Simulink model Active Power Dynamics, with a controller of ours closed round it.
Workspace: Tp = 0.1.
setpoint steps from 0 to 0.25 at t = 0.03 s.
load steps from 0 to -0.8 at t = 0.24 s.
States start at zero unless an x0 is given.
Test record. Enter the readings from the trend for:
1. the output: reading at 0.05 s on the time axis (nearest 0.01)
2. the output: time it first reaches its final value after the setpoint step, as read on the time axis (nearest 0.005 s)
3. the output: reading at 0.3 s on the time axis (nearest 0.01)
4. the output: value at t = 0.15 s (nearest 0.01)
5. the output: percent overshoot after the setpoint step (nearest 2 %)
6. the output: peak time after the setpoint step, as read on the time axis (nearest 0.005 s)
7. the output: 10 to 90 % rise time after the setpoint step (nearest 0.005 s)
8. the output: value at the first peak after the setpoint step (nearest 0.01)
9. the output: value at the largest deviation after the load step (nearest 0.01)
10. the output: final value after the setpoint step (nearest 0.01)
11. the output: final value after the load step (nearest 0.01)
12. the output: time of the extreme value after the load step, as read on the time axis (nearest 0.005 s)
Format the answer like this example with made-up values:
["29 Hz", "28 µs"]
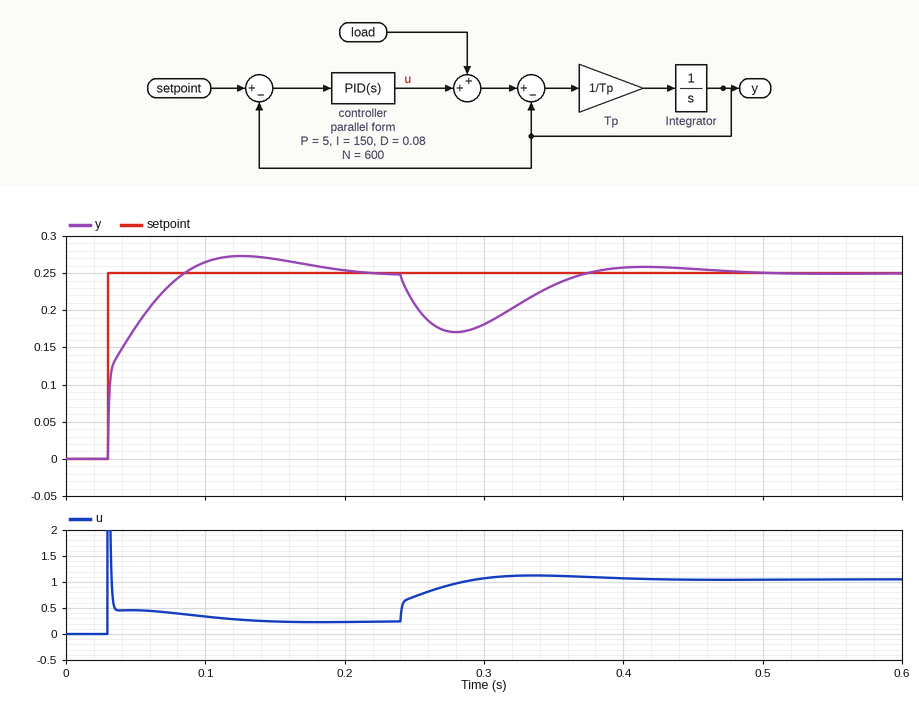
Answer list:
["0.18", "0.085 s", "0.18", "0.27", "10 %", "0.125 s", "0.040 s", "0.27", "0.17", "0.25", "0.25", "0.280 s"]
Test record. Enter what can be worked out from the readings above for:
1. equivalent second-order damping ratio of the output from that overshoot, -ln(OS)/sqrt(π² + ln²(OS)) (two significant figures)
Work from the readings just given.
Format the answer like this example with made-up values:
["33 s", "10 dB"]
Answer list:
["0.59"]
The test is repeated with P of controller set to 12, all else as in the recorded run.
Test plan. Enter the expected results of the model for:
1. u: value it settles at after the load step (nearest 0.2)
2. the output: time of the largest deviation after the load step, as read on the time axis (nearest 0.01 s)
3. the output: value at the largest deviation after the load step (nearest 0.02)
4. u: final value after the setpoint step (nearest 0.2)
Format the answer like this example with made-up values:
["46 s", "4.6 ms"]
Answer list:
["1.0", "0.27 s", "0.20", "0.2"]
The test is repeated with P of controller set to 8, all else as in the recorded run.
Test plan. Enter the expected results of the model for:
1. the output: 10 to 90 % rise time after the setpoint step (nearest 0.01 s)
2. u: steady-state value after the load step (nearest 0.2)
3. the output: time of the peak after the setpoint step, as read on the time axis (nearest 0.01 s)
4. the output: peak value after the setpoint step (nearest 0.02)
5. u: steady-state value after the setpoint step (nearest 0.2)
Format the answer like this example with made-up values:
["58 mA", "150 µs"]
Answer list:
["0.03 s", "1.0", "0.12 s", "0.26", "0.2"]
